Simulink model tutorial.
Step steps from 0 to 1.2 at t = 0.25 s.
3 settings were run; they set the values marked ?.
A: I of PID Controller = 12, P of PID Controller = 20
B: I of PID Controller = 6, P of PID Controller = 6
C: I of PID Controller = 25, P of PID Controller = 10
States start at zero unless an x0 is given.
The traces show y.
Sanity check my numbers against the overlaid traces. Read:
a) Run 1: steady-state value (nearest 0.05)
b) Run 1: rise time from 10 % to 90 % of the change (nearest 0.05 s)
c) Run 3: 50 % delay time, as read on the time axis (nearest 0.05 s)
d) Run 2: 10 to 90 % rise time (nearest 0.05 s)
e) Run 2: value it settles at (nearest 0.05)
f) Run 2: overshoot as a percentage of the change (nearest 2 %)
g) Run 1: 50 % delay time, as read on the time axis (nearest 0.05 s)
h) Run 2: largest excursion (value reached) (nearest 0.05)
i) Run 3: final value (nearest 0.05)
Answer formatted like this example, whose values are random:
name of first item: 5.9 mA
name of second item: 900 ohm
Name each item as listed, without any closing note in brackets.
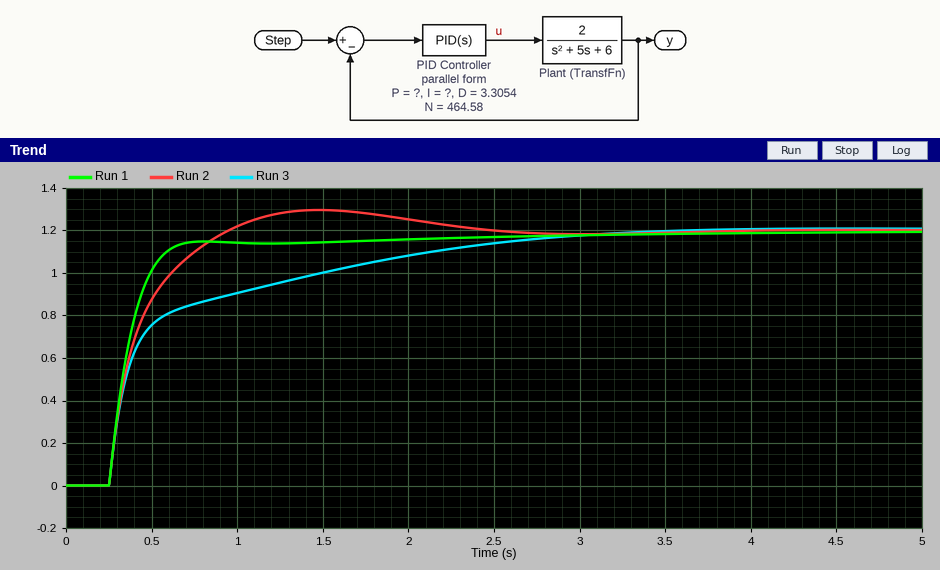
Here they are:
Run 1: steady-state value: 1.20
Run 1: rise time from 10 % to 90 % of the change: 0.30 s
Run 3: 50 % delay time, as read on the time axis: 0.40 s
Run 2: 10 to 90 % rise time: 0.45 s
Run 2: value it settles at: 1.20
Run 2: overshoot as a percentage of the change: 8 %
Run 1: 50 % delay time, as read on the time axis: 0.35 s
Run 2: largest excursion (value reached): 1.30
Run 3: final value: 1.20
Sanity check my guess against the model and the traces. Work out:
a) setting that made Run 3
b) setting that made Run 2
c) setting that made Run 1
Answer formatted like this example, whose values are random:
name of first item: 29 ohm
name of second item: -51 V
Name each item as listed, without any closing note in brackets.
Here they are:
setting that made Run 3: B
setting that made Run 2: C
setting that made Run 1: A
